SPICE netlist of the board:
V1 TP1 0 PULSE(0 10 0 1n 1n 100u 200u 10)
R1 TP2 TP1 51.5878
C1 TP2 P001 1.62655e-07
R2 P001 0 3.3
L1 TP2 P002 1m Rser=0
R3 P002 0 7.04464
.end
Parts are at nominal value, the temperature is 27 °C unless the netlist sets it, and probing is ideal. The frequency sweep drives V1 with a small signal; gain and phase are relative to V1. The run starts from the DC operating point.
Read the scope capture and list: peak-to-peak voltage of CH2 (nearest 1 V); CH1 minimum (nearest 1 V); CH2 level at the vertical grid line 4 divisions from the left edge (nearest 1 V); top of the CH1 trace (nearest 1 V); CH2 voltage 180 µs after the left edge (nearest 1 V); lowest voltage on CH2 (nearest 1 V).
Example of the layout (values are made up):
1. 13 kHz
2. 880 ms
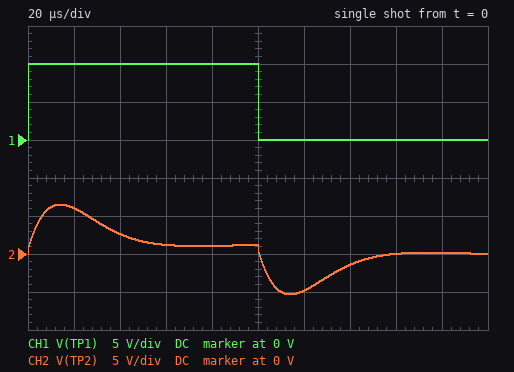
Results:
1. 12 V
2. 0 V
3. 1 V
4. 10 V
5. 0 V
6. -5 V
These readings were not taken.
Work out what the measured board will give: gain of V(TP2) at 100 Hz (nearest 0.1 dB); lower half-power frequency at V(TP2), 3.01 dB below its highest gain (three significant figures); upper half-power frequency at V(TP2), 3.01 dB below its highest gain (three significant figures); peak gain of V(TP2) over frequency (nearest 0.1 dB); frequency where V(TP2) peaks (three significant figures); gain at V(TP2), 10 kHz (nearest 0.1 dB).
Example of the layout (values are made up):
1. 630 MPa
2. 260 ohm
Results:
1. -18.4 dB
2. 6.35 kHz
3. 25.9 kHz
4. -0.7 dB
5. 12.9 kHz
6. -1.2 dB
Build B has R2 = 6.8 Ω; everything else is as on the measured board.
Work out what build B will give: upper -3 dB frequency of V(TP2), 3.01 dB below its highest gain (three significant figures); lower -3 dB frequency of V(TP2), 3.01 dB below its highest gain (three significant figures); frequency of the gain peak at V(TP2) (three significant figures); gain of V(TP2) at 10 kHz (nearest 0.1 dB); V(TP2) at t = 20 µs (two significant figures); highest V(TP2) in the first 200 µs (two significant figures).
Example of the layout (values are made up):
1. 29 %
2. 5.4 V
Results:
1. 25.3 kHz
2. 6.17 kHz
3. 12.5 kHz
4. -1.3 dB
5. 5.9 V
6. 6.3 V
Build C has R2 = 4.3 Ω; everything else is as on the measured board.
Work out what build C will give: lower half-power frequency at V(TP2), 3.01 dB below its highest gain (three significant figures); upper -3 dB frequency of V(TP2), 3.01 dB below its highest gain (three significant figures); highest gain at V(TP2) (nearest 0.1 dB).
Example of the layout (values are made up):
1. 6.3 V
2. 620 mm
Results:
1. 6.29 kHz
2. 25.7 kHz
3. -0.8 dB
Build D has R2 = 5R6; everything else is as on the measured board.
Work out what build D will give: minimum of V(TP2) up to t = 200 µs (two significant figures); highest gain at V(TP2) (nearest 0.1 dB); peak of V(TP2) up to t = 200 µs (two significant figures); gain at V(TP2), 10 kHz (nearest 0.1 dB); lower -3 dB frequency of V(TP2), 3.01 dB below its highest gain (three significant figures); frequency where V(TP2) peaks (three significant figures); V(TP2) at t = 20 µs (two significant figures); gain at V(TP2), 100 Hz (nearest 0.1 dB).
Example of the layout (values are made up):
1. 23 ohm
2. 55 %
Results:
1. -5.2 V
2. -0.9 dB
3. 6.4 V
4. -1.3 dB
5. 6.23 kHz
6. 12.6 kHz
7. 5.9 V
8. -18.4 dB
